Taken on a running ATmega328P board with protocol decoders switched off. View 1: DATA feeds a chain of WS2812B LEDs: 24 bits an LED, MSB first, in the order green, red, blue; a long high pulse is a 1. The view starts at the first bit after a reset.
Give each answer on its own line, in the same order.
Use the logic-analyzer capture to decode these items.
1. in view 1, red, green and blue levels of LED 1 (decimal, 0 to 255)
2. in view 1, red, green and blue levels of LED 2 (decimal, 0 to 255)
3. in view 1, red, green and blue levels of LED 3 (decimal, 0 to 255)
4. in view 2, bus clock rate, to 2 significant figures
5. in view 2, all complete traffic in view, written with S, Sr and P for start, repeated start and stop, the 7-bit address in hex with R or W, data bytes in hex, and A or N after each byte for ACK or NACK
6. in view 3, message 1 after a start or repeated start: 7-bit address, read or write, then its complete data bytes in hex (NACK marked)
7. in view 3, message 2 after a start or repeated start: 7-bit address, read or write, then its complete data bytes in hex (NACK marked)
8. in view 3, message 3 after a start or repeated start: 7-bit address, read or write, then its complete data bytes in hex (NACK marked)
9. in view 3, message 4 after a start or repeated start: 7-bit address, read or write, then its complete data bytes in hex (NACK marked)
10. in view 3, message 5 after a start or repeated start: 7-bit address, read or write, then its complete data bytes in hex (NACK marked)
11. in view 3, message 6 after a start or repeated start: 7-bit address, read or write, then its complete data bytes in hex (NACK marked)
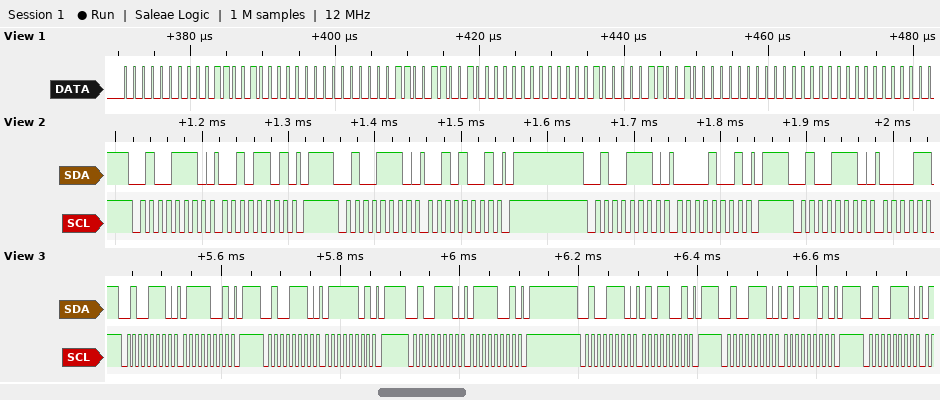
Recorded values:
50, 0, 0
50, 3, 0
50, 8, 0
100 kHz
S 27W A 2D A P S 27W A 29 A P S 27W A 09 A P S 27W A
0x27 write: 79
0x27 write: 7D
0x27 write: 79
0x27 write: 59
0x27 write: 5D
0x27 write
